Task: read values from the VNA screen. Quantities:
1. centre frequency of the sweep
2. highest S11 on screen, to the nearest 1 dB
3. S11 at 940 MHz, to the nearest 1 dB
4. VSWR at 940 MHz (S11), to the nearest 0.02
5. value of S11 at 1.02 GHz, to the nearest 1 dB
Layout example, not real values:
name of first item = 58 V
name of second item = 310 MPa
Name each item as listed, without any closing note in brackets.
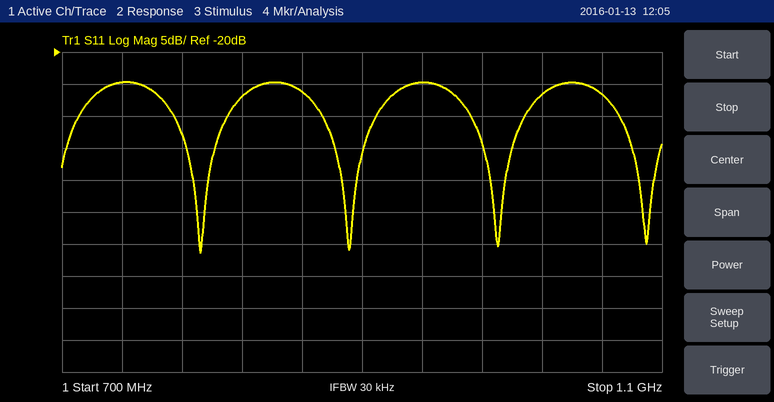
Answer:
centre frequency of the sweep = 900 MHz
highest S11 on screen, to the nearest 1 dB = -25 dB
S11 at 940 MHz, to the nearest 1 dB = -25 dB
VSWR at 940 MHz (S11), to the nearest 0.02 = 1.12
value of S11 at 1.02 GHz, to the nearest 1 dB = -27 dB
